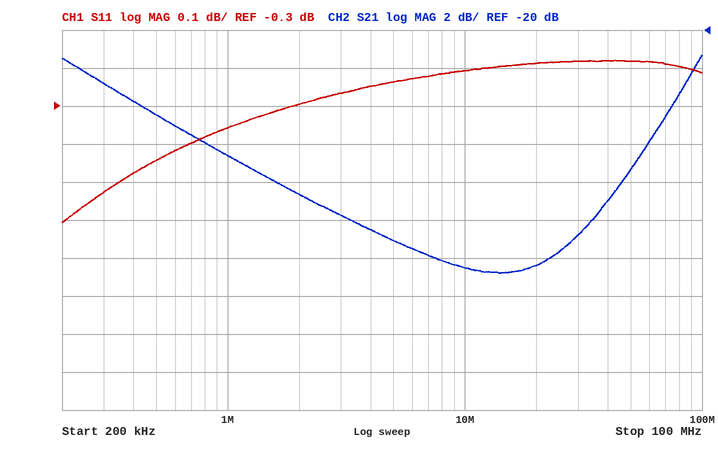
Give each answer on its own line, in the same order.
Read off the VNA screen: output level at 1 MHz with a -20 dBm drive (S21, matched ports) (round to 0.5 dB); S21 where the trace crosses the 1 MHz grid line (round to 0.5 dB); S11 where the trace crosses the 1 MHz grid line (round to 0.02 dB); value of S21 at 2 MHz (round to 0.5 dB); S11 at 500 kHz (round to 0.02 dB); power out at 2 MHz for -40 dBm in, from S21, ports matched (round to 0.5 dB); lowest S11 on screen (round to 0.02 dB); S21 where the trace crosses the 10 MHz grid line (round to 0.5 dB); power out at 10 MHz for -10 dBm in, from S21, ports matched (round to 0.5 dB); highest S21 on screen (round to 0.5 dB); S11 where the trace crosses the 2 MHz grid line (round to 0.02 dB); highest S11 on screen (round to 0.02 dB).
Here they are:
-46.5 dBm
-26.5 dB
-0.36 dB
-28.5 dB
-0.44 dB
-68.5 dBm
-0.60 dB
-32.5 dB
-42.5 dBm
-21.5 dB
-0.30 dB
-0.18 dB
